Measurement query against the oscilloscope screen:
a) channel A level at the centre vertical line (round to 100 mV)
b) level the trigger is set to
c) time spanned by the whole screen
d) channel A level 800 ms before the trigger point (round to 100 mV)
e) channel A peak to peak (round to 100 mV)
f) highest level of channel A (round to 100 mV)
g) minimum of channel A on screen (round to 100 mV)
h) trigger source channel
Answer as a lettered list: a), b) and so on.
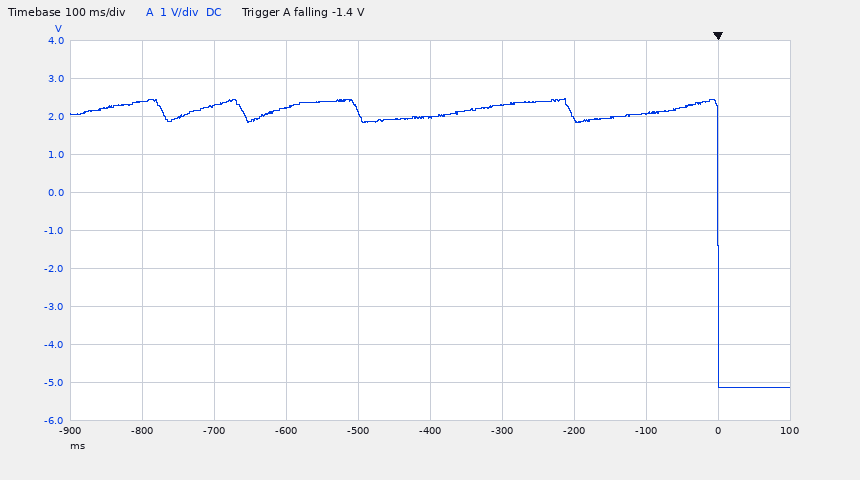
a) 2.0 V
b) -1.4 V
c) 1 s
d) 2.4 V
e) 7.6 V
f) 2.5 V
g) -5.1 V
h) channel A
